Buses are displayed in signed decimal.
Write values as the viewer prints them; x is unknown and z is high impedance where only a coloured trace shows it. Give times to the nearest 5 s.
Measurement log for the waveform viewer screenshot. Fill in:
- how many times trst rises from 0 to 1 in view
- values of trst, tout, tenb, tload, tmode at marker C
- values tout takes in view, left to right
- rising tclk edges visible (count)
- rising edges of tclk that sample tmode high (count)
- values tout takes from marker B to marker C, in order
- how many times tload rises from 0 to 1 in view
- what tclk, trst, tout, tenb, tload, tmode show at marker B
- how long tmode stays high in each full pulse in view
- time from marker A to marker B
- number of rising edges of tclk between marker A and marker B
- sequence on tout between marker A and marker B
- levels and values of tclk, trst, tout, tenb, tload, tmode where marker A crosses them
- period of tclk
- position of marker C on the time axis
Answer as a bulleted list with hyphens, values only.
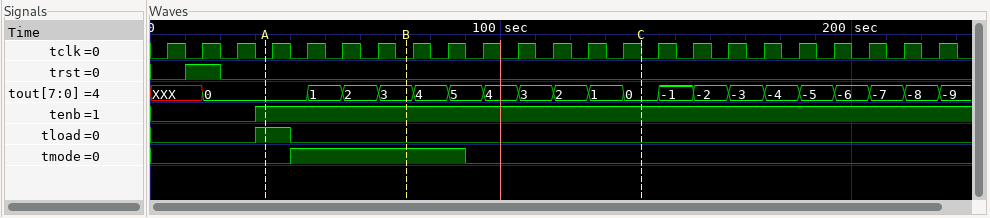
- 1
- trst=0, tout=0, tenb=1, tload=0, tmode=0
- XXX, 0, 1, 2, 3, 4, 5, 4, 3, 2, 1, 0, -1, -2, -3, -4, -5, -6, -7, -8, -9
- 23
- 5
- 3, 4, 5, 4, 3, 2, 1, 0
- 1
- tclk=0, trst=0, tout=3, tenb=1, tload=0, tmode=1
- 50 s
- 40 s
- 4
- 0, 1, 2, 3
- tclk=0, trst=0, tout=0, tenb=1, tload=1, tmode=0
- 10 s
- 140 s
